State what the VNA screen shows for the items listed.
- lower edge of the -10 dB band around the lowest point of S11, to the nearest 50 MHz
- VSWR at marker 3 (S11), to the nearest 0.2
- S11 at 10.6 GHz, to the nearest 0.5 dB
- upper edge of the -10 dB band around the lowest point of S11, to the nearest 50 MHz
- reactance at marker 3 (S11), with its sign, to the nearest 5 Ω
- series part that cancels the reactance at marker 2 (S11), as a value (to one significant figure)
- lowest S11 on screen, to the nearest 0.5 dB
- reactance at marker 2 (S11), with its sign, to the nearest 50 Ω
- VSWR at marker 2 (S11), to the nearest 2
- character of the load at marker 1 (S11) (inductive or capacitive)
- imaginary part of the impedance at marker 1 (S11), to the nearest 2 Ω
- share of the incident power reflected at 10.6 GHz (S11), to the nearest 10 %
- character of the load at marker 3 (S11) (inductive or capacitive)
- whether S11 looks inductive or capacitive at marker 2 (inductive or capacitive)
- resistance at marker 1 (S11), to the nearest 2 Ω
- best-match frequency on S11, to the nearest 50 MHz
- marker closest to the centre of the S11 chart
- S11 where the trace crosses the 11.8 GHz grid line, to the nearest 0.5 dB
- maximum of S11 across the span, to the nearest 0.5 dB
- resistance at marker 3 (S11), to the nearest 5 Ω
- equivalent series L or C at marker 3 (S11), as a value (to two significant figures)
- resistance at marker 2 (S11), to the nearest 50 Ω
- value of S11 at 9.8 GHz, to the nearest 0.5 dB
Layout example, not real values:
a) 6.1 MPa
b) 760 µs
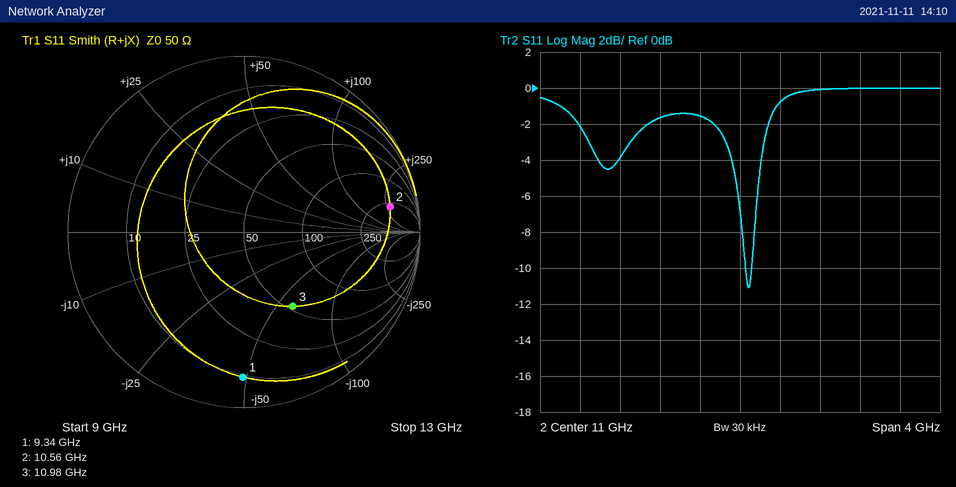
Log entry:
a) 11.05 GHz
b) 3.0
c) -1.5 dB
d) 11.10 GHz
e) -60 Ω
f) 50 fF
g) -11.0 dB
h) +300 Ω
i) 12
j) capacitive
k) -48 Ω
l) 70 %
m) capacitive
n) inductive
o) 10 Ω
p) 11.10 GHz
q) marker 3
r) 0.0 dB
s) 0.0 dB
t) 55 Ω
u) 240 fF
v) 300 Ω
w) -4.0 dB
